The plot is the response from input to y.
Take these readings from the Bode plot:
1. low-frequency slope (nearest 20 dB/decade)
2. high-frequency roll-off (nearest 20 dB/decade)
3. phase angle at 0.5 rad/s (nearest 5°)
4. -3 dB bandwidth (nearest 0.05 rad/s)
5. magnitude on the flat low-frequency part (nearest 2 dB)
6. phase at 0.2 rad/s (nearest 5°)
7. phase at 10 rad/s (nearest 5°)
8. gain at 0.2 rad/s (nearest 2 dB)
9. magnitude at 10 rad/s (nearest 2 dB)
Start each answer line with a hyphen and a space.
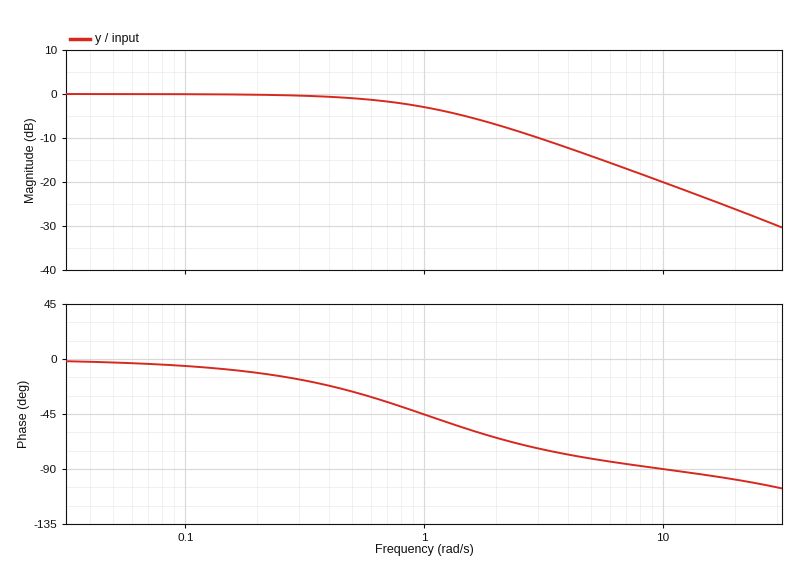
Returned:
- 0 dB/decade
- -20 dB/decade
- -25°
- 1.00 rad/s
- 0 dB
- -10°
- -90°
- 0 dB
- -20 dB
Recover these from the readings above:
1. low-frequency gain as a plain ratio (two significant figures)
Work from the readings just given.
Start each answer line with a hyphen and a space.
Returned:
- 1.0
